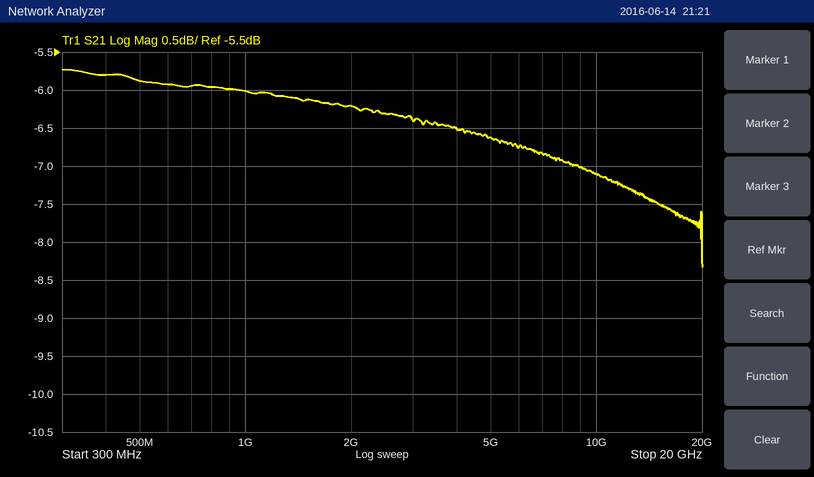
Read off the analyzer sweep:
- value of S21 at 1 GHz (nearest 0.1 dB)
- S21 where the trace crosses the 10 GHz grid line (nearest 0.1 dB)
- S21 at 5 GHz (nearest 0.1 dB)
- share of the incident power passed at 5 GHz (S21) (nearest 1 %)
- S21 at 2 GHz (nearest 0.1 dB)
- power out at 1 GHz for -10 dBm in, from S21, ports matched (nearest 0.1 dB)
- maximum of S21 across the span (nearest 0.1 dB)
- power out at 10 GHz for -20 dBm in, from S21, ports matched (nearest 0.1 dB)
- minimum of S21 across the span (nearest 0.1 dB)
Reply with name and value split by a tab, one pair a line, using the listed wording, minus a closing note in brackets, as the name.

value of S21 at 1 GHz	-6.0 dB
S21 where the trace crosses the 10 GHz grid line	-7.1 dB
S21 at 5 GHz	-6.6 dB
share of the incident power passed at 5 GHz (S21)	22 %
S21 at 2 GHz	-6.2 dB
power out at 1 GHz for -10 dBm in, from S21, ports matched	-16.0 dBm
maximum of S21 across the span	-5.7 dB
power out at 10 GHz for -20 dBm in, from S21, ports matched	-27.1 dBm
minimum of S21 across the span	-8.3 dB
